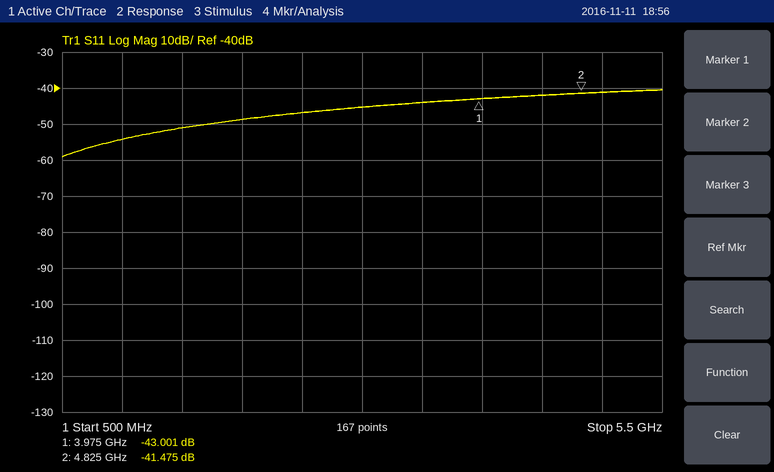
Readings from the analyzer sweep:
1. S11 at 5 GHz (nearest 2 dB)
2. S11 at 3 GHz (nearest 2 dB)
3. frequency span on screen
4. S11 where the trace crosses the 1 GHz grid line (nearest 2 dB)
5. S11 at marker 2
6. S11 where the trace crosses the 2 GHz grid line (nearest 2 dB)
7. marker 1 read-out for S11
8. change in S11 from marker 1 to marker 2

-42 dB
-46 dB
5 GHz
-54 dB
-41.475 dB
-48 dB
-43.001 dB
1.526 dB
